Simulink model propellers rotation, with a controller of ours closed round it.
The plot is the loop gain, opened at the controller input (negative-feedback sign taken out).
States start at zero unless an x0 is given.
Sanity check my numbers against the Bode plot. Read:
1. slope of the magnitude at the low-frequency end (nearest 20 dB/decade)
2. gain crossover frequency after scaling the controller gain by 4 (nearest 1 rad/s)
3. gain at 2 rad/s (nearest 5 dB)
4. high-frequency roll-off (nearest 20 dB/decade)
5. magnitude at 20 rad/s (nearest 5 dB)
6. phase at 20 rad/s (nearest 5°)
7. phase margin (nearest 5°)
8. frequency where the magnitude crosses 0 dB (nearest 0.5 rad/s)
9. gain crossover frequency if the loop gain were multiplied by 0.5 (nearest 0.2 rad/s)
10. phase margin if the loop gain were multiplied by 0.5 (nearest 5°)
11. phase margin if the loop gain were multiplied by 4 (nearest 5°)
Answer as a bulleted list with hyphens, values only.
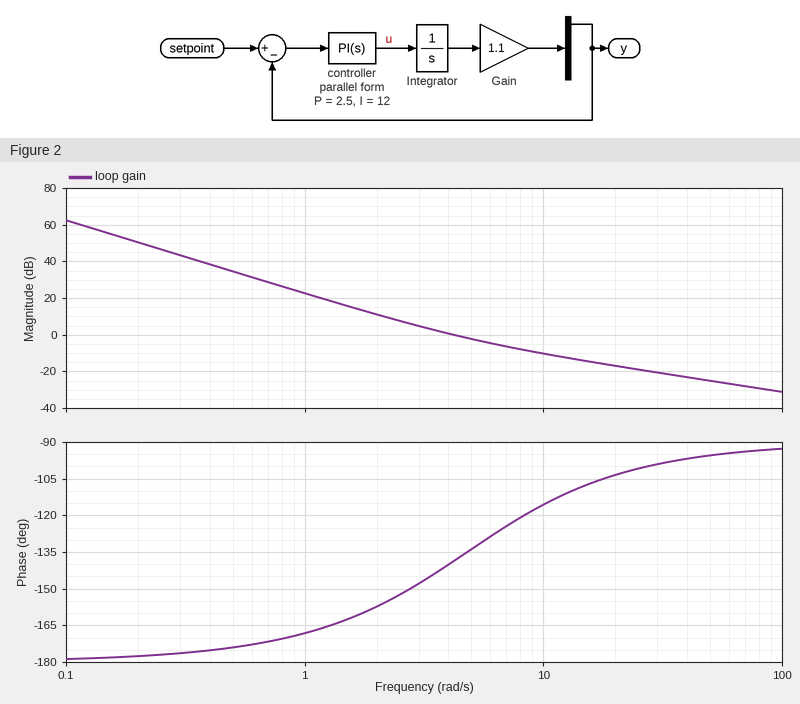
- -40 dB/decade
- 12 rad/s
- 10 dB
- -20 dB/decade
- -15 dB
- -105°
- 40°
- 4.0 rad/s
- 2.8 rad/s
- 30°
- 70°
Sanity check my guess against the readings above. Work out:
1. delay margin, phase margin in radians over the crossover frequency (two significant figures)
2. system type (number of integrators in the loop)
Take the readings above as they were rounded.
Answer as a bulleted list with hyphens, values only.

- 0.17 s
- 2
